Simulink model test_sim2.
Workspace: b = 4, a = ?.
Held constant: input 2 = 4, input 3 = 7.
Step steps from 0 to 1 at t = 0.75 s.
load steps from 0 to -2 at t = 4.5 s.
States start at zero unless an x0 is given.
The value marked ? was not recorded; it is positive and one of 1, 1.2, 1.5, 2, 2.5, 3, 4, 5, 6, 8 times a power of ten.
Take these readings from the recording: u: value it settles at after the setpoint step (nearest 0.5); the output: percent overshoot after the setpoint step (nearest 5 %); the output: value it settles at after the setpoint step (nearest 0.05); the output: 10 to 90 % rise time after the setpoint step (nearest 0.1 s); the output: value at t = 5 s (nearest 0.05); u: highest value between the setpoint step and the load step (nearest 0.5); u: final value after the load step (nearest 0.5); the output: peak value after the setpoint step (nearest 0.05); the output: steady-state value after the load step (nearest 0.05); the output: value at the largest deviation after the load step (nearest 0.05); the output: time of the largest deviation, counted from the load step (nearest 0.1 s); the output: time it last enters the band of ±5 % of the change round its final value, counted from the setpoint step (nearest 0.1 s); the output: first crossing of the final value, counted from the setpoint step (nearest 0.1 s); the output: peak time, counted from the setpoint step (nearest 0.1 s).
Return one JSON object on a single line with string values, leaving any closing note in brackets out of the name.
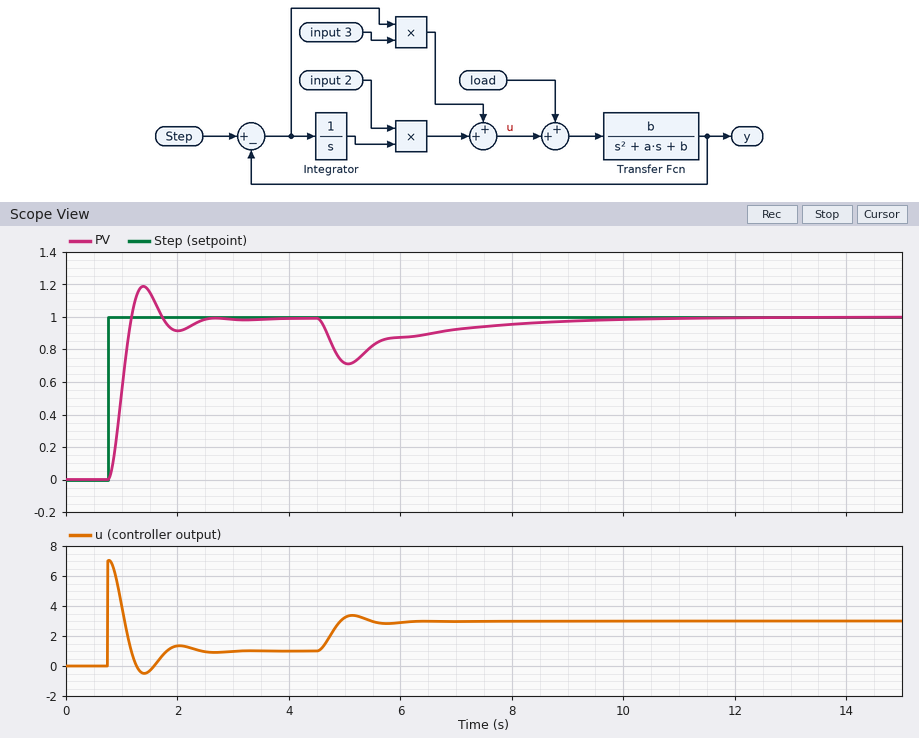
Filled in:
{"u: value it settles at after the setpoint step": "1.0", "the output: percent overshoot after the setpoint step": "20 %", "the output: value it settles at after the setpoint step": "1.00", "the output: 10 to 90 % rise time after the setpoint step": "0.3 s", "the output: value at t = 5 s": "0.70", "u: highest value between the setpoint step and the load step": "7.0", "u: final value after the load step": "3.0", "the output: peak value after the setpoint step": "1.20", "the output: steady-state value after the load step": "1.00", "the output: value at the largest deviation after the load step": "0.70", "the output: time of the largest deviation, counted from the load step": "0.6 s", "the output: time it last enters the band of ±5 % of the change round its final value, counted from the setpoint step": "1.5 s", "the output: first crossing of the final value, counted from the setpoint step": "0.4 s", "the output: peak time, counted from the setpoint step": "0.6 s"}
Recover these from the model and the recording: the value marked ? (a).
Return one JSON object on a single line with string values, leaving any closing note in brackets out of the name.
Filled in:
{"the value marked ?": "5"}
